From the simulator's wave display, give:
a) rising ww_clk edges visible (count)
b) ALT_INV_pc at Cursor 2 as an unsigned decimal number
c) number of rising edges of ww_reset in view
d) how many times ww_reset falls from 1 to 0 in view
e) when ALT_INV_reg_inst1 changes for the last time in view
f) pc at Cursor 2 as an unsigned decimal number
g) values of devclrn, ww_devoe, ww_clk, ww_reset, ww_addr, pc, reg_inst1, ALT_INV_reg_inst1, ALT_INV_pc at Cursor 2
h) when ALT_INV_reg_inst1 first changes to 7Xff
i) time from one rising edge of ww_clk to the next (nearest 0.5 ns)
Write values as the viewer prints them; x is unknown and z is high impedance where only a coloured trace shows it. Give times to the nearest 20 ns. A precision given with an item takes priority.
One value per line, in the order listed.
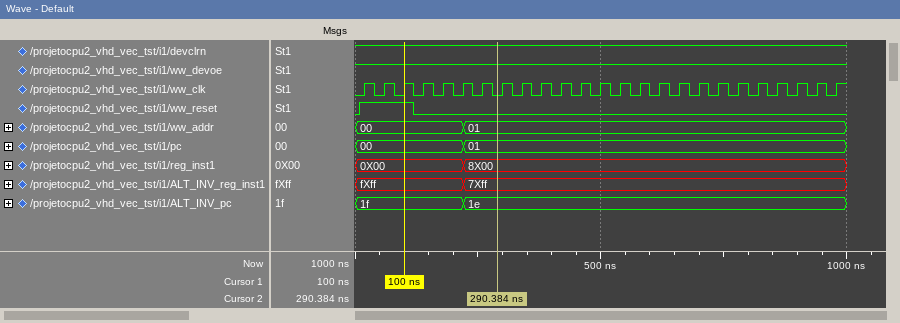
25
30
1
1
220 ns
1
devclrn=1, ww_devoe=1, ww_clk=0, ww_reset=0, ww_addr=01, pc=01, reg_inst1=8X00, ALT_INV_reg_inst1=7Xff, ALT_INV_pc=1e
220 ns
40 ns
